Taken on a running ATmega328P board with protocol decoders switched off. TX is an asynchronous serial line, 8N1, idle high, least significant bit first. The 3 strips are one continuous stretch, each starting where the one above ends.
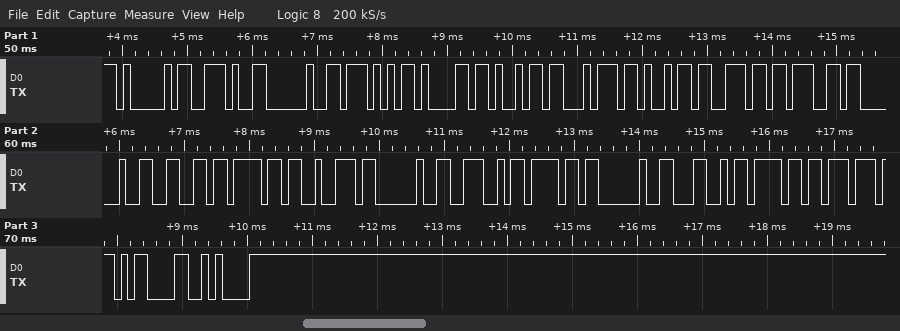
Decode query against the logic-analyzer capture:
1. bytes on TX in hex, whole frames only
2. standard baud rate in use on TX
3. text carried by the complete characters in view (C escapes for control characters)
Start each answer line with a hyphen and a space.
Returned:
- 41 2E 20 57 61 69 74 69 6E 67 20 66 6F 72 20 4E 6F 20 4C 6F 77 0D 0A
- 9600 baud
- "A. Waiting for No Low\r\n"
